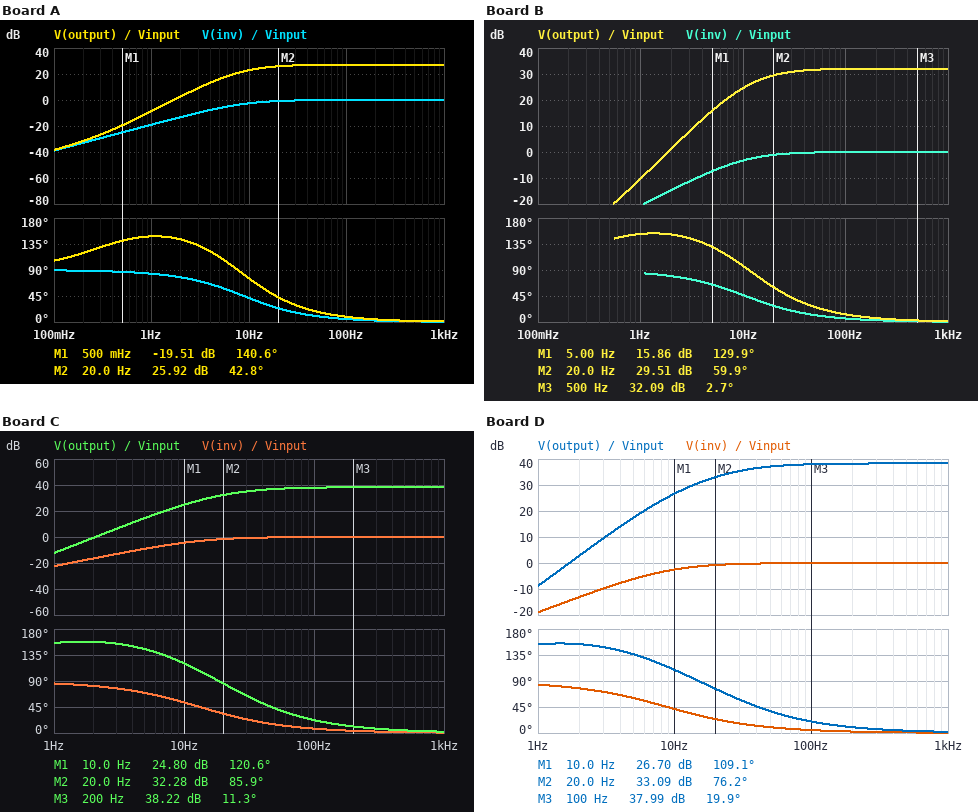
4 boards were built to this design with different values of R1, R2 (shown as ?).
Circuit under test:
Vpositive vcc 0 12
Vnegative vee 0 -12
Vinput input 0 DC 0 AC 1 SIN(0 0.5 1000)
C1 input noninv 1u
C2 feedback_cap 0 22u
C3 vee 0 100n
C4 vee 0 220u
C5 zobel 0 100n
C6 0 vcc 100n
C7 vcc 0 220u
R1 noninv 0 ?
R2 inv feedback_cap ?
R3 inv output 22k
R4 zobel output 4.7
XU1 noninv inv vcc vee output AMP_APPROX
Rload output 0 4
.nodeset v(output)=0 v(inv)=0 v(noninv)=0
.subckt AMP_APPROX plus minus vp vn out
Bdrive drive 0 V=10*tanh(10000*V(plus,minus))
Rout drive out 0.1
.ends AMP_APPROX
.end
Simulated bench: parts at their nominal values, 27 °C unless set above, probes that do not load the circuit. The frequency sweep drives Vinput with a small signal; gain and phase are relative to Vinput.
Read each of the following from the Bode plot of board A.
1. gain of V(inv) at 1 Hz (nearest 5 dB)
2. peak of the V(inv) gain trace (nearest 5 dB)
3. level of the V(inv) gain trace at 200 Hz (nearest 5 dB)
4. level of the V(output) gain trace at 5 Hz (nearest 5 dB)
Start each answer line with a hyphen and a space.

- -20 dB
- 0 dB
- 0 dB
- 15 dB
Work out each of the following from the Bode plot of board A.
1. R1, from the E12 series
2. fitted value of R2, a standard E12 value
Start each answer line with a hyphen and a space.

- 18 kΩ
- 1 kΩ
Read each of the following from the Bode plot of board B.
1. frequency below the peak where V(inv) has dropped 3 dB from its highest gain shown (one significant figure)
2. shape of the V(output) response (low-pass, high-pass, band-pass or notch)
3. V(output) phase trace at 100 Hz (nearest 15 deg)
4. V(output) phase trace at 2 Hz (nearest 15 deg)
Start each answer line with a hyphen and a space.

- 10 Hz
- high-pass
- 15 deg
- 150 deg
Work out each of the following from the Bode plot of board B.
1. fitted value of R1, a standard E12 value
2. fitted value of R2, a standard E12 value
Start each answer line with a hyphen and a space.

- 15 kΩ
- 560 Ω
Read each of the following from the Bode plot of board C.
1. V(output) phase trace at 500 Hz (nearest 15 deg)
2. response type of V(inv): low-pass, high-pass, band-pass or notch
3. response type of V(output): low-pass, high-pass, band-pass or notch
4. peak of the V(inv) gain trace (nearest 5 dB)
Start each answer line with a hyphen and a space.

- 0 deg
- high-pass
- high-pass
- 0 dB
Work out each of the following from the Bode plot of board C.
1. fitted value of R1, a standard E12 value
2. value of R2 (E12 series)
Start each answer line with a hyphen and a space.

- 12 kΩ
- 270 Ω
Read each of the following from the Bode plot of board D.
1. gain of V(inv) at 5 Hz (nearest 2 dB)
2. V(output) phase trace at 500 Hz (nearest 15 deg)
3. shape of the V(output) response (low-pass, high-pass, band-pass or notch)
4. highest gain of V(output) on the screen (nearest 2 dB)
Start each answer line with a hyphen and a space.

- -6 dB
- 0 deg
- high-pass
- 38 dB
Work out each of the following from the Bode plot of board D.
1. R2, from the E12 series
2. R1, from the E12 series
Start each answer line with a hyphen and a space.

- 270 Ω
- 18 kΩ
